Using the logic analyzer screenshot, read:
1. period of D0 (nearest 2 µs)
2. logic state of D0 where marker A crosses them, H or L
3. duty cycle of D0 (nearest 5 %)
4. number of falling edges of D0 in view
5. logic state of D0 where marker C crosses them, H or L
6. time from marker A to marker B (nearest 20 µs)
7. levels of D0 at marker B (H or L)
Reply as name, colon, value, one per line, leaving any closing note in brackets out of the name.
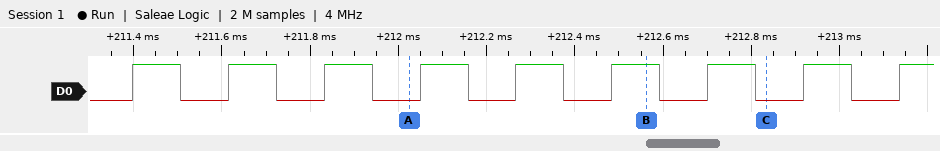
period of D0: 218 µs
logic state of D0 where marker A crosses them, H or L: D0=L
duty cycle of D0: 50 %
number of falling edges of D0 in view: 8
logic state of D0 where marker C crosses them, H or L: D0=L
time from marker A to marker B: 540 µs
levels of D0 at marker B: D0=H
